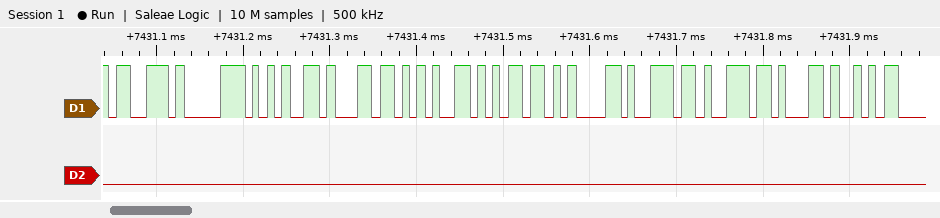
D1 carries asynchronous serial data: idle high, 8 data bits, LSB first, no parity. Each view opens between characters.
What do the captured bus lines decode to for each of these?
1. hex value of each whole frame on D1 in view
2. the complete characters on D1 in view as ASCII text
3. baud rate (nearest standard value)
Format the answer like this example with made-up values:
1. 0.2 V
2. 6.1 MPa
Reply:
1. 73, 70, 65, 6C, 65, 6D, 61, 6E, 6E, 2C
2. "spelemann,"
3. 115200 baud
